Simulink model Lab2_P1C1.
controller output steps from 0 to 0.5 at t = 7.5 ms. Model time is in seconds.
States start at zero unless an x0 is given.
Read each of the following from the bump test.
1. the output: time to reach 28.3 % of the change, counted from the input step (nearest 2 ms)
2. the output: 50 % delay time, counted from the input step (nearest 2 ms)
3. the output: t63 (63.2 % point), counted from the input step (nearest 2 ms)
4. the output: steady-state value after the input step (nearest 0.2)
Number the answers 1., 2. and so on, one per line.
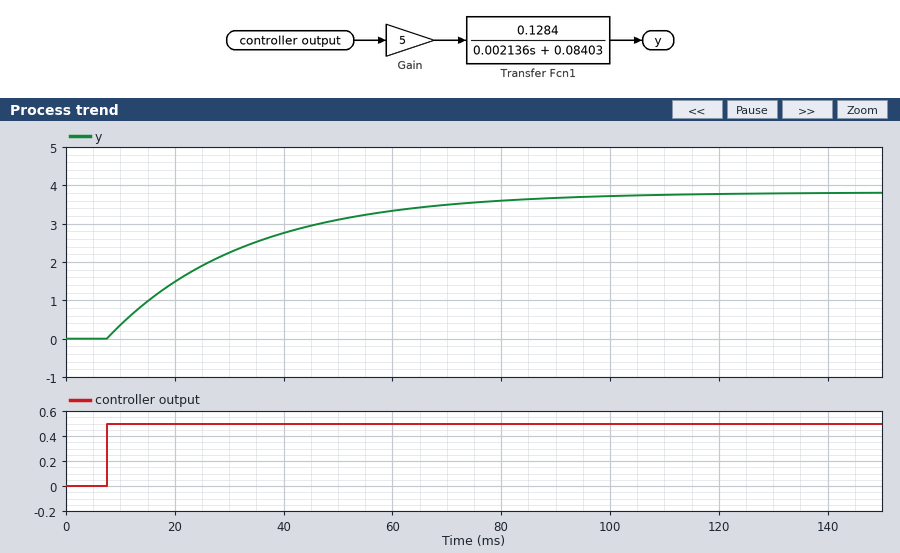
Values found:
1. 8 ms
2. 18 ms
3. 26 ms
4. 3.8
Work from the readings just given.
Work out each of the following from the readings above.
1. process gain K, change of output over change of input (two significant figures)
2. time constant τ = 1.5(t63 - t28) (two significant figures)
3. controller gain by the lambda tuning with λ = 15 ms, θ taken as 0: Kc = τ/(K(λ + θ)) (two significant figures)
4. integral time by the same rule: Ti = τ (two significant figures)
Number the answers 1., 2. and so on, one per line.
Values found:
1. 7.6
2. 27 ms
3. 0.24
4. 27 ms
